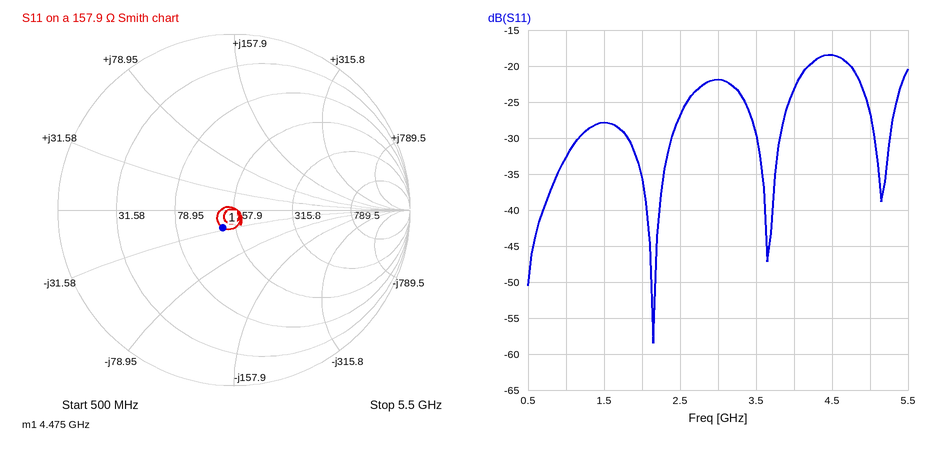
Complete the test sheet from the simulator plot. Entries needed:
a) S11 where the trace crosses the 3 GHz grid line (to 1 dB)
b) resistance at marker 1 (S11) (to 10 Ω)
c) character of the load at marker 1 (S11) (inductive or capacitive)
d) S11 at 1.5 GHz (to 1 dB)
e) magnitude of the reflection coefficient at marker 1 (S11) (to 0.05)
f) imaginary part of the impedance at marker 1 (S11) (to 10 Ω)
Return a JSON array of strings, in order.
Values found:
["-22 dB", "140 Ω", "capacitive", "-28 dB", "0.10", "-30 Ω"]
